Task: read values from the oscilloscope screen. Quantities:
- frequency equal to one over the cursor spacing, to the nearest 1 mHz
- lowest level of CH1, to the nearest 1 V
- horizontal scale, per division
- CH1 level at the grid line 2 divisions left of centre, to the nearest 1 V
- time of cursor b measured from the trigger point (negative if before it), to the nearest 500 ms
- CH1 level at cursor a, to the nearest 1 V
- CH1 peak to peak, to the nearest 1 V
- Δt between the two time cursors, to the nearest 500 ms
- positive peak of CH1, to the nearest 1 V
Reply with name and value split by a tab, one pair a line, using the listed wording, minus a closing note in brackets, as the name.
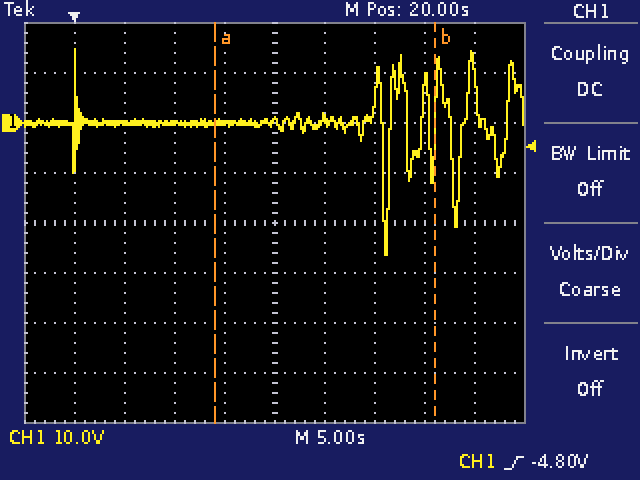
frequency equal to one over the cursor spacing, to the nearest 1 mHz	45 mHz
lowest level of CH1, to the nearest 1 V	-26 V
horizontal scale, per division	5 s
CH1 level at the grid line 2 divisions left of centre, to the nearest 1 V	0 V
time of cursor b measured from the trigger point (negative if before it), to the nearest 500 ms	+36.0 s
CH1 level at cursor a, to the nearest 1 V	0 V
CH1 peak to peak, to the nearest 1 V	41 V
Δt between the two time cursors, to the nearest 500 ms	22.0 s
positive peak of CH1, to the nearest 1 V	15 V
